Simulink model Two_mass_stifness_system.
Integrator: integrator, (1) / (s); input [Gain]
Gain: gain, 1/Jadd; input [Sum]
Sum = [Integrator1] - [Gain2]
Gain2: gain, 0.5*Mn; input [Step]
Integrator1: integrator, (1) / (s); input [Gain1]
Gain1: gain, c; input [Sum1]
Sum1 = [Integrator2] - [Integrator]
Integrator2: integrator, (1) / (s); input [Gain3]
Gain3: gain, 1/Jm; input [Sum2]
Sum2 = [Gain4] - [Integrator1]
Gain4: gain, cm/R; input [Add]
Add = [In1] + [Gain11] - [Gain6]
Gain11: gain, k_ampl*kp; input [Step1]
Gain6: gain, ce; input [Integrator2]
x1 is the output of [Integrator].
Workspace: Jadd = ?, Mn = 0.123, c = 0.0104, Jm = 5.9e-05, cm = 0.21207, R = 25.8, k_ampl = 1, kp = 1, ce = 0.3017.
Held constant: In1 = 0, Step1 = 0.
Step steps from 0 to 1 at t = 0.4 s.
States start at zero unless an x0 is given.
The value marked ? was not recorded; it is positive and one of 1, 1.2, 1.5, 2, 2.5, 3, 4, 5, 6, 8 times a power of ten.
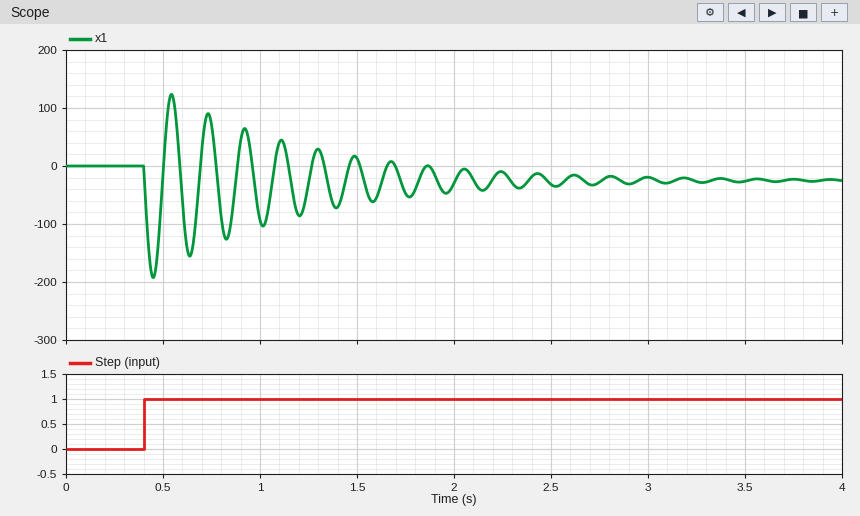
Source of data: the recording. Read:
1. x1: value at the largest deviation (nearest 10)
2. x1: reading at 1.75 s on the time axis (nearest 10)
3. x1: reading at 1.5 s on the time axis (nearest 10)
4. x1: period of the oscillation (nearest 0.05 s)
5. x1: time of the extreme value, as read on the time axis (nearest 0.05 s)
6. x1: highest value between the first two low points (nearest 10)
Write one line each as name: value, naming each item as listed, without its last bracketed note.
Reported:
x1: value at the largest deviation: -190
x1: reading at 1.75 s on the time axis: -50
x1: reading at 1.5 s on the time axis: 10
x1: period of the oscillation: 0.20 s
x1: time of the extreme value, as read on the time axis: 0.45 s
x1: highest value between the first two low points: 120
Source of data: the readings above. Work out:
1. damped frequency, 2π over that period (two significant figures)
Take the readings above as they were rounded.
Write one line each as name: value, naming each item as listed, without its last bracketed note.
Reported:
damped frequency, 2π over that period: 31 rad/s
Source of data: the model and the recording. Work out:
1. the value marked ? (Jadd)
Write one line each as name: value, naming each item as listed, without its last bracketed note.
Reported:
the value marked ?: 1e-05
